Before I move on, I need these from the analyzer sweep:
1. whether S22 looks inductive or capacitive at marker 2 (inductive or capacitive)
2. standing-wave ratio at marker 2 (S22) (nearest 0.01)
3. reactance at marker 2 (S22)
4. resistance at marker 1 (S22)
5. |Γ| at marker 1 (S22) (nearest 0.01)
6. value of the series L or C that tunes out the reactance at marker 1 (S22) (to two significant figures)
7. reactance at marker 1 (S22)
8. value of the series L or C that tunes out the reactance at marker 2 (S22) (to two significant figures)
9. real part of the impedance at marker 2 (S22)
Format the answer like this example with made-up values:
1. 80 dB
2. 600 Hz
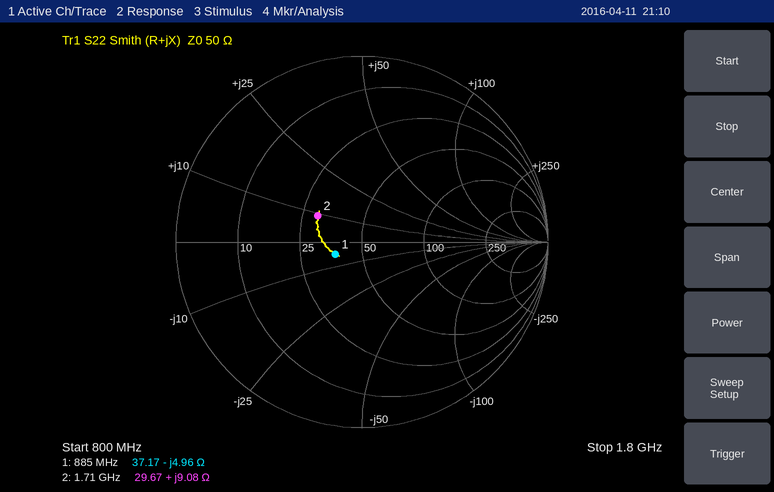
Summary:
1. inductive
2. 1.77
3. +9.08 Ω
4. 37.17 Ω
5. 0.16
6. 890 pH
7. -4.96 Ω
8. 10 pF
9. 29.67 Ω
